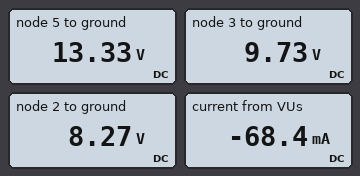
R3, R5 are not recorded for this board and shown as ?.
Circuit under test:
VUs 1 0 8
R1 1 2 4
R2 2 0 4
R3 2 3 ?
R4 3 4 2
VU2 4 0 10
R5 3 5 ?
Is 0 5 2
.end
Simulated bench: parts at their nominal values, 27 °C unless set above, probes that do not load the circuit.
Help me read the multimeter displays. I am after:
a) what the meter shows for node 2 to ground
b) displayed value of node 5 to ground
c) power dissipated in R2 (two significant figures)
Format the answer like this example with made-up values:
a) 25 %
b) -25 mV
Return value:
a) 8.27 V
b) 13.33 V
c) 17 W
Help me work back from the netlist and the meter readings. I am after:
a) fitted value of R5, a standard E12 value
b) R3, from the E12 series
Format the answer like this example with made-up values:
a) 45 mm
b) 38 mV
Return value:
a) 1.8 Ω
b) 0.68 Ω
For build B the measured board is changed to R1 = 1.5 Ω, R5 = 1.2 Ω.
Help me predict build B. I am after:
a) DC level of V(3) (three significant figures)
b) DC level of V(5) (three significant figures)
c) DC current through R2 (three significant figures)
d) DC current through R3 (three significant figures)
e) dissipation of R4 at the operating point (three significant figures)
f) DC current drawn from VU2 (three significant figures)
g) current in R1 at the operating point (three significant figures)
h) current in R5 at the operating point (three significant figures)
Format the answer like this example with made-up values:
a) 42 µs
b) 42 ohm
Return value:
a) 9.66 V
b) 12.1 V
c) 2.05 A
d) 2.17 A
e) 57.6 mW
f) 170 mA
g) 123 mA
h) 2.00 A
